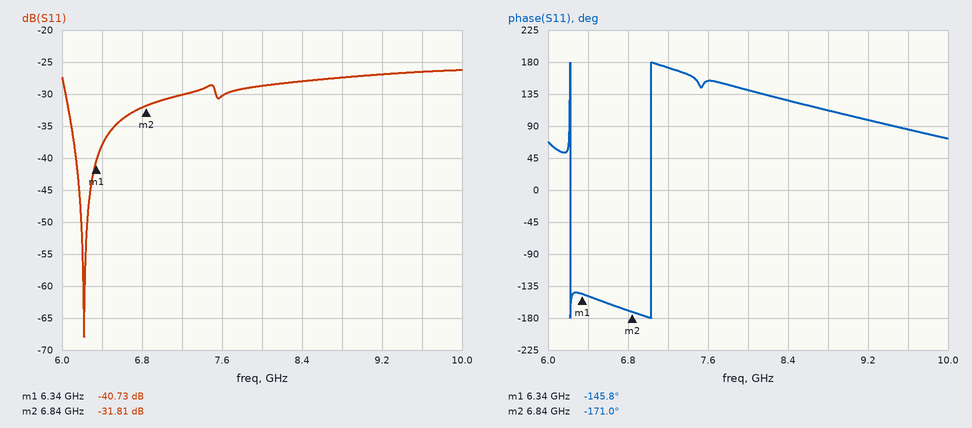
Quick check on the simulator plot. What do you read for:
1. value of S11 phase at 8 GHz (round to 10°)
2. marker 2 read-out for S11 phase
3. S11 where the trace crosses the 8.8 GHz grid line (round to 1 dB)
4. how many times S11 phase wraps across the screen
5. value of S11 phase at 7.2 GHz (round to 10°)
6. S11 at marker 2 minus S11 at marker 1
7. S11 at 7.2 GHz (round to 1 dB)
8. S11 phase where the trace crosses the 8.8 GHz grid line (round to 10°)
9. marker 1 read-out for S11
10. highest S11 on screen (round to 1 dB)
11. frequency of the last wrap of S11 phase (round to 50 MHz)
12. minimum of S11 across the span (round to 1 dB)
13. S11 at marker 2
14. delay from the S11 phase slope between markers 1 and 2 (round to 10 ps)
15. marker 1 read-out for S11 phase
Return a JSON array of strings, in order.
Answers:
["140°", "-171.0°", "-27 dB", "2", "170°", "8.92 dB", "-30 dB", "110°", "-40.73 dB", "-26 dB", "7.05 GHz", "-68 dB", "-31.81 dB", "140 ps", "-145.8°"]
